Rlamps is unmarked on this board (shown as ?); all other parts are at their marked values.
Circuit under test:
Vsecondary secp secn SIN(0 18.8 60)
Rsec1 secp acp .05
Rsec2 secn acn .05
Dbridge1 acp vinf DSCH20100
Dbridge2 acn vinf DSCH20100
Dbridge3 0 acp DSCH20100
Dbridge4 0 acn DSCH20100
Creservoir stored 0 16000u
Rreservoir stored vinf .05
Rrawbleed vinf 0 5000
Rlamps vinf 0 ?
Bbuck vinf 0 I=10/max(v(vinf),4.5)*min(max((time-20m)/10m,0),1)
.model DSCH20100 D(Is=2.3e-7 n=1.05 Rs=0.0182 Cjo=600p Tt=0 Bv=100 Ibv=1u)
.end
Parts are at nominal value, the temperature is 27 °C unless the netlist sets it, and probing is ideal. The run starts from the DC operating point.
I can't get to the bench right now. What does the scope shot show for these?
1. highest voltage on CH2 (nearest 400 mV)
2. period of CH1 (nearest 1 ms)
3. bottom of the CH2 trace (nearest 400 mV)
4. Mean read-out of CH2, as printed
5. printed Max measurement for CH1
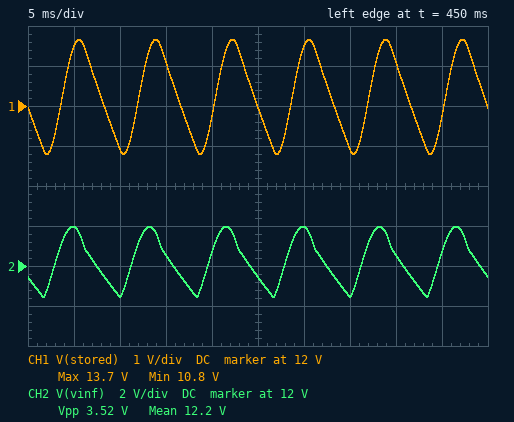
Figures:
14.0 V
8 ms
10.4 V
12.2 V
13.7 V
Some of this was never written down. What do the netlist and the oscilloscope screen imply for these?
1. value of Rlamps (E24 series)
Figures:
1.2 Ω
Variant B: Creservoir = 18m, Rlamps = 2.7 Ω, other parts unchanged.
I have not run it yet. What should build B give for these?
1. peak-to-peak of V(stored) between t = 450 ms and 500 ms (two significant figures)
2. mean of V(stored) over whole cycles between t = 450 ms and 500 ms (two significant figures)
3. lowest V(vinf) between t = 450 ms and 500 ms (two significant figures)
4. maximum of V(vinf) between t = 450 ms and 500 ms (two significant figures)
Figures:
1.6 V
14 V
13 V
15 V
